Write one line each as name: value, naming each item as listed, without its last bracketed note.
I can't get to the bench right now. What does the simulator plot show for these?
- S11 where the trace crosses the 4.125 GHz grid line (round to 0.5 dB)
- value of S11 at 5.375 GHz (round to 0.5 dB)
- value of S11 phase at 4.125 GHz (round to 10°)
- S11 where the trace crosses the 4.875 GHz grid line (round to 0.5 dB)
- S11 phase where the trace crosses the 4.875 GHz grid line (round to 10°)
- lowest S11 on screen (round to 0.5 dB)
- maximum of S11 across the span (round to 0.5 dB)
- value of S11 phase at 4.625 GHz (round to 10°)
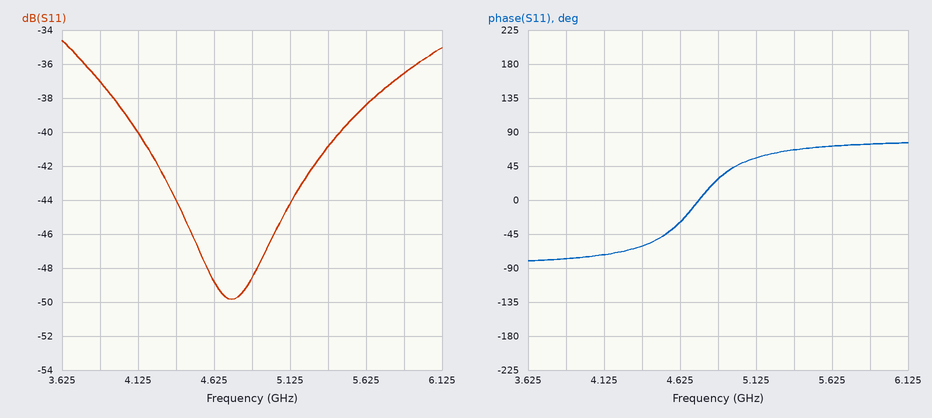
S11 where the trace crosses the 4.125 GHz grid line: -40.0 dB
value of S11 at 5.375 GHz: -41.0 dB
value of S11 phase at 4.125 GHz: -70°
S11 where the trace crosses the 4.875 GHz grid line: -48.5 dB
S11 phase where the trace crosses the 4.875 GHz grid line: 30°
lowest S11 on screen: -50.0 dB
maximum of S11 across the span: -34.5 dB
value of S11 phase at 4.625 GHz: -30°
